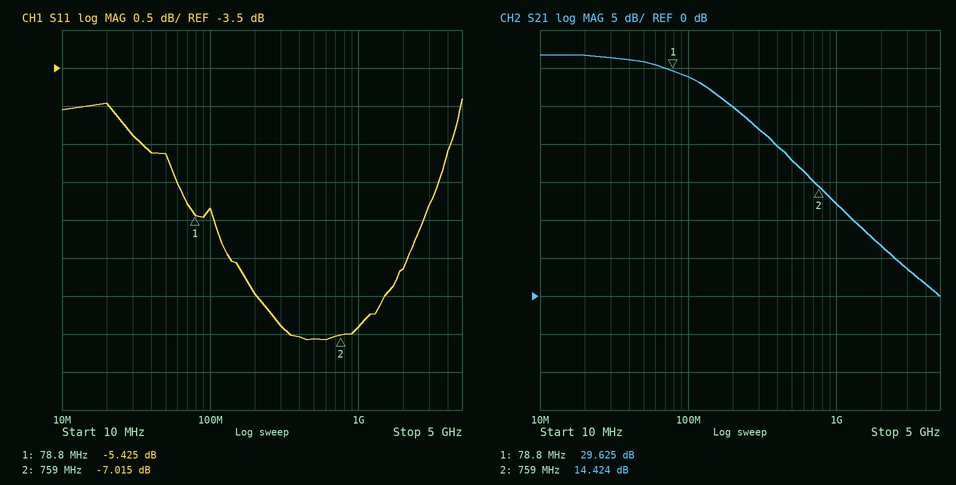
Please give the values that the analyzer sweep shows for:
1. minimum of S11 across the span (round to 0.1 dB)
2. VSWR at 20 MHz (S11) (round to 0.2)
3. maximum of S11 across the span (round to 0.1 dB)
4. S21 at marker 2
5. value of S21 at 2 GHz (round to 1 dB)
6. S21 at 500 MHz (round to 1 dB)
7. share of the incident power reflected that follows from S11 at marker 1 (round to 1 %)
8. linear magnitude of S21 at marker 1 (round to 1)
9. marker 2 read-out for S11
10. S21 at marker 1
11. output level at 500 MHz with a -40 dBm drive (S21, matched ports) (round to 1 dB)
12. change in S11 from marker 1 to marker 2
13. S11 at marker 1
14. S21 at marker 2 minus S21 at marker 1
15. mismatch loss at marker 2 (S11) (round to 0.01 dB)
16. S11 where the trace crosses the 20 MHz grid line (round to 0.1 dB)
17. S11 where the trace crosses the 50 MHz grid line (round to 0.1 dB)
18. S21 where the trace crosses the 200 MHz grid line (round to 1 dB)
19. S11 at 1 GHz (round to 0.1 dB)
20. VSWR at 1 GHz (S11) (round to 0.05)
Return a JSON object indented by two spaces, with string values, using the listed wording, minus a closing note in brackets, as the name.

{
  "minimum of S11 across the span": "-7.1 dB",
  "VSWR at 20 MHz (S11)": "4.4",
  "maximum of S11 across the span": "-3.9 dB",
  "S21 at marker 2": "14.424 dB",
  "value of S21 at 2 GHz": "7 dB",
  "S21 at 500 MHz": "18 dB",
  "share of the incident power reflected that follows from S11 at marker 1": "29 %",
  "linear magnitude of S21 at marker 1": "30",
  "marker 2 read-out for S11": "-7.015 dB",
  "S21 at marker 1": "29.625 dB",
  "output level at 500 MHz with a -40 dBm drive (S21, matched ports)": "-22 dBm",
  "change in S11 from marker 1 to marker 2": "-1.590 dB",
  "S11 at marker 1": "-5.425 dB",
  "S21 at marker 2 minus S21 at marker 1": "-15.201 dB",
  "mismatch loss at marker 2 (S11)": "0.96 dB",
  "S11 where the trace crosses the 20 MHz grid line": "-4.0 dB",
  "S11 where the trace crosses the 50 MHz grid line": "-4.6 dB",
  "S21 where the trace crosses the 200 MHz grid line": "25 dB",
  "S11 at 1 GHz": "-6.9 dB",
  "VSWR at 1 GHz (S11)": "2.65"
}
